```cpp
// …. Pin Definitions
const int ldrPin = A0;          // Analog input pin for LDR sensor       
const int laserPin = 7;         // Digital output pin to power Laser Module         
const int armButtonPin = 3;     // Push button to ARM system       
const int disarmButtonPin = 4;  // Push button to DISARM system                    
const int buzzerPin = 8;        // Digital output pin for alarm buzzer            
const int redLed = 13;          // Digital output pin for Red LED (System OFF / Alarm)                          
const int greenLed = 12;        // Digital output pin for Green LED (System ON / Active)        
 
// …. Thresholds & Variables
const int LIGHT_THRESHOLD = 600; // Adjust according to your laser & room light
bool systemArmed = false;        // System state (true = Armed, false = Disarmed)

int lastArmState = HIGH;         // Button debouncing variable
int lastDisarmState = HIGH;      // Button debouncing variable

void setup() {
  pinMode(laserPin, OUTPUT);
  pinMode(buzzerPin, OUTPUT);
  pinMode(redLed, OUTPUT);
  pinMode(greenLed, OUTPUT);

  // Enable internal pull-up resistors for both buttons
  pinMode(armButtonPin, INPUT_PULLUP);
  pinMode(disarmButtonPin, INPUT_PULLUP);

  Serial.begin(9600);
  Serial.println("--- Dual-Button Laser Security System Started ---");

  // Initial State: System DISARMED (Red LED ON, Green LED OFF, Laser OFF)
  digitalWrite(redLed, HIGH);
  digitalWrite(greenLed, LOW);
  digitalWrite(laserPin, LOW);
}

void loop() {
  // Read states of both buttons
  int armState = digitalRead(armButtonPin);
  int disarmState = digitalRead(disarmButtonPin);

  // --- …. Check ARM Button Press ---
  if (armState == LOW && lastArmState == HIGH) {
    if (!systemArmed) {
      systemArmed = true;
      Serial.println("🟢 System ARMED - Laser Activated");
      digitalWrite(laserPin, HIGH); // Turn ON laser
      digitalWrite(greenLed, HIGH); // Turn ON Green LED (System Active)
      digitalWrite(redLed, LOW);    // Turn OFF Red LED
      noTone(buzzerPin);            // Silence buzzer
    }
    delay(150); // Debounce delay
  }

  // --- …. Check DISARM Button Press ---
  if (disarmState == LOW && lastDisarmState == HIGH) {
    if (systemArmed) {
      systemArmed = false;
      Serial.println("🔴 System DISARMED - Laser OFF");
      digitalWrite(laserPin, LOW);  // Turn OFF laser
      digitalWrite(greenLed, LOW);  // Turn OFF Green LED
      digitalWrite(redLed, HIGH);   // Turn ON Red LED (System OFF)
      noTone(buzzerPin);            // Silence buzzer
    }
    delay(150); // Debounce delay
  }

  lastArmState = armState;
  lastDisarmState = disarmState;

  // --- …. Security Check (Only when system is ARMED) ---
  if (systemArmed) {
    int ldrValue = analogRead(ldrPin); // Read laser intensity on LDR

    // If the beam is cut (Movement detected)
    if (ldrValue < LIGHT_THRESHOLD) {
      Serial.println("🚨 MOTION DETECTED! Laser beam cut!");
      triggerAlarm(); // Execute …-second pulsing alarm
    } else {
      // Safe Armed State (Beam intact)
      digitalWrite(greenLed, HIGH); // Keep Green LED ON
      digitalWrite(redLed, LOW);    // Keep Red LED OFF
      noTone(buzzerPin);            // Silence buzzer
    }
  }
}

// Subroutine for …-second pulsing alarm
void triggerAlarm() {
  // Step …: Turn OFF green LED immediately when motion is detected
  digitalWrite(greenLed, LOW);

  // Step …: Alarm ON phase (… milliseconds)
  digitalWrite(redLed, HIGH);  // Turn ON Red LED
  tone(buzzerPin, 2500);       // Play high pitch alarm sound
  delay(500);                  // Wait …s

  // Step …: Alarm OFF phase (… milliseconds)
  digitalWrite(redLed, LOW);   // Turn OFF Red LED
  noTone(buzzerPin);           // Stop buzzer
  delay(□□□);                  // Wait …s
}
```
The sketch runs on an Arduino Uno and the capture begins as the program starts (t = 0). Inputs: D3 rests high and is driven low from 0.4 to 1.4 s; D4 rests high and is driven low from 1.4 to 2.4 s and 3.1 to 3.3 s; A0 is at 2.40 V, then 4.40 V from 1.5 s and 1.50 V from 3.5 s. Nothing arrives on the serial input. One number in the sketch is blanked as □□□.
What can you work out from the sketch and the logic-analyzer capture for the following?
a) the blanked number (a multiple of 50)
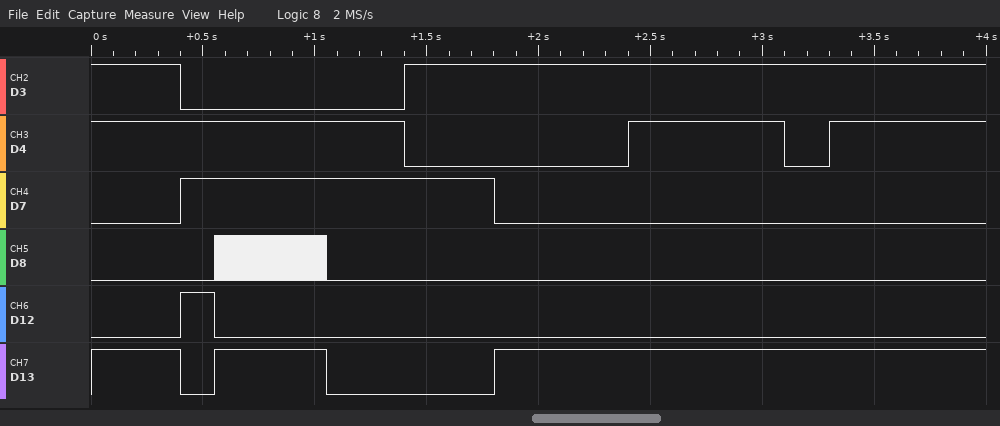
750
